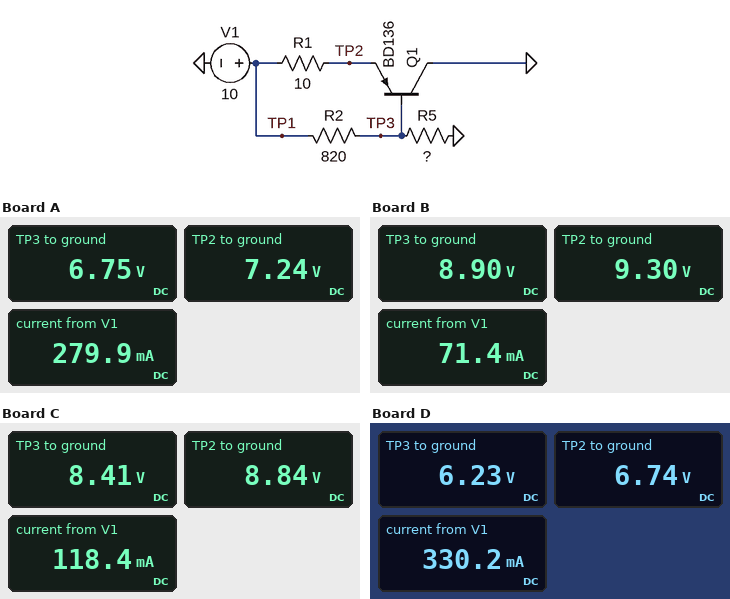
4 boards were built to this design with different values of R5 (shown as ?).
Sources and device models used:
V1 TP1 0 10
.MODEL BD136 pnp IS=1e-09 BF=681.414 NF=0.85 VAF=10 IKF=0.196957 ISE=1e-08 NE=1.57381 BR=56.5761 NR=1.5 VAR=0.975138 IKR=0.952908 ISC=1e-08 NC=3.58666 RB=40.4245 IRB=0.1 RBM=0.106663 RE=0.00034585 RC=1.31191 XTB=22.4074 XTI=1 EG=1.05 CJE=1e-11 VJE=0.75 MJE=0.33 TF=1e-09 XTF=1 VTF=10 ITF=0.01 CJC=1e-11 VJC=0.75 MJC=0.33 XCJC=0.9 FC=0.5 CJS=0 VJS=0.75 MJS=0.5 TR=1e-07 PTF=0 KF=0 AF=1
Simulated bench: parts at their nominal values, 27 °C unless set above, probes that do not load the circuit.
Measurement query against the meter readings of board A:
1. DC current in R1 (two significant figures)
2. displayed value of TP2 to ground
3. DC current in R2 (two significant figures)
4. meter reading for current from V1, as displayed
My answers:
280 mA
7.24 V
4.0 mA
279.9 mA
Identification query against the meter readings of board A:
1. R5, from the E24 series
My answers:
1.3 kΩ
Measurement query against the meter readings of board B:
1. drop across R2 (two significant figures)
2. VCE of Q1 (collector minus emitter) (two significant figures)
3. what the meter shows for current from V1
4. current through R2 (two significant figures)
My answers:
1.1 V
-9.3 V
71.4 mA
1.3 mA
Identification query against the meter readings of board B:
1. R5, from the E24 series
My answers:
5.6 kΩ
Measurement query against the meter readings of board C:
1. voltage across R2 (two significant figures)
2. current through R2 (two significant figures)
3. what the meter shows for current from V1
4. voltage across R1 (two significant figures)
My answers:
1.6 V
1.9 mA
118.4 mA
1.2 V
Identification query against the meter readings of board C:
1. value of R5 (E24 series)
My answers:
3.6 kΩ
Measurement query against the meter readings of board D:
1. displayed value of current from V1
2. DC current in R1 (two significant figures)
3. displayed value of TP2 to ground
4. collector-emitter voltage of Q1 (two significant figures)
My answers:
330.2 mA
330 mA
6.74 V
-6.7 V
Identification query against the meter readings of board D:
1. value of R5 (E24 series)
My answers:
1 kΩ
